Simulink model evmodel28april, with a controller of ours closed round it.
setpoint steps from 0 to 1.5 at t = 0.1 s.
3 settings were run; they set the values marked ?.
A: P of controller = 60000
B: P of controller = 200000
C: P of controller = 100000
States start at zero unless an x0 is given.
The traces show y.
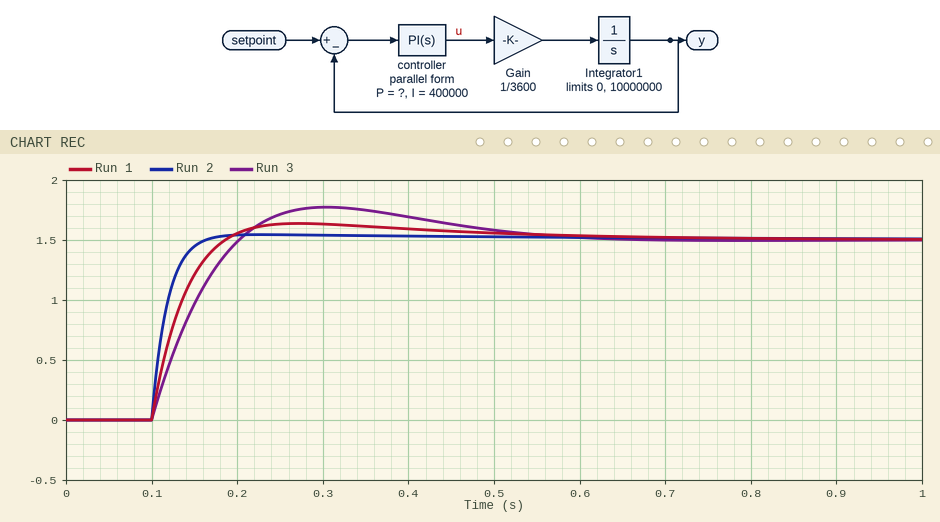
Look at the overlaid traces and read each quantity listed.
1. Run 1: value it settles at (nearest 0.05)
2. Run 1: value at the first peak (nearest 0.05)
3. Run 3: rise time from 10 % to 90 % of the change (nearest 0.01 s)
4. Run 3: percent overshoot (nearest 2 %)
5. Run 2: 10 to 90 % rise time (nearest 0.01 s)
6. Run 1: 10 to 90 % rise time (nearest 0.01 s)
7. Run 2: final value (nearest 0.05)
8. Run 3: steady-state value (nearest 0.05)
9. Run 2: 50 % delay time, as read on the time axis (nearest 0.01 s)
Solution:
1.50
1.65
0.08 s
18 %
0.04 s
0.06 s
1.50
1.50
0.11 s
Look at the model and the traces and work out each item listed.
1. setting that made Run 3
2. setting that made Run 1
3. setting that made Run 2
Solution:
A
C
B
